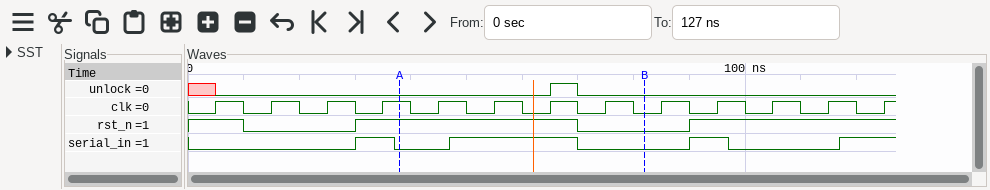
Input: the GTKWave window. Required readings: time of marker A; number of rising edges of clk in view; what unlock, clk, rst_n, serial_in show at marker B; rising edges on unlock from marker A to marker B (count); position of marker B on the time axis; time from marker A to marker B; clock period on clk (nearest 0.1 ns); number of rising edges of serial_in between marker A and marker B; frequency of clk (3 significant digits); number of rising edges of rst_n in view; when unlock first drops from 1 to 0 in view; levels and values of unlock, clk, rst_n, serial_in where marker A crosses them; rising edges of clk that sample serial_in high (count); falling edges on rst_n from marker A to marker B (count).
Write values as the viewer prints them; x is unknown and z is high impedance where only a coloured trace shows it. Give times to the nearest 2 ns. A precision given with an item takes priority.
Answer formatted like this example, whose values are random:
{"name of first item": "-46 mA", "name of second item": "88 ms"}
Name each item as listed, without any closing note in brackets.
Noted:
{"time of marker A": "38 ns", "number of rising edges of clk in view": "13", "what unlock, clk, rst_n, serial_in show at marker B": "unlock=0, clk=0, rst_n=0, serial_in=0", "rising edges on unlock from marker A to marker B": "1", "position of marker B on the time axis": "82 ns", "time from marker A to marker B": "44 ns", "clock period on clk": "10 ns", "number of rising edges of serial_in between marker A and marker B": "1", "frequency of clk": "100 MHz", "number of rising edges of rst_n in view": "2", "when unlock first drops from 1 to 0 in view": "70 ns", "levels and values of unlock, clk, rst_n, serial_in where marker A crosses them": "unlock=0, clk=1, rst_n=1, serial_in=0", "rising edges of clk that sample serial_in high": "5", "falling edges on rst_n from marker A to marker B": "1"}
